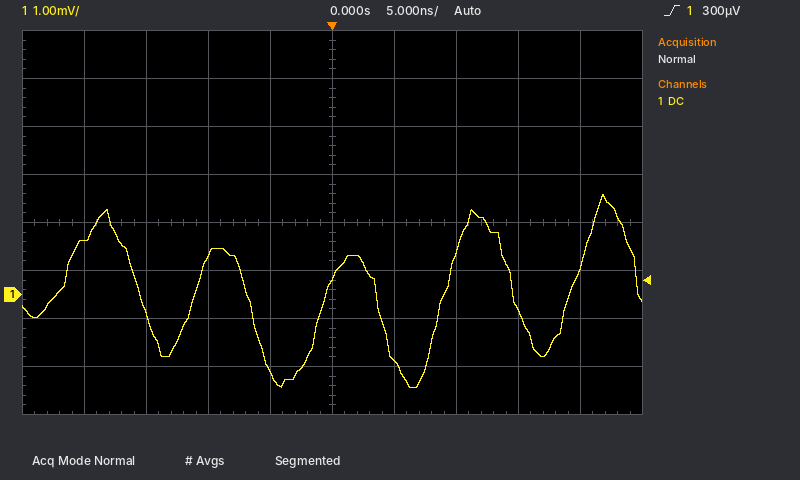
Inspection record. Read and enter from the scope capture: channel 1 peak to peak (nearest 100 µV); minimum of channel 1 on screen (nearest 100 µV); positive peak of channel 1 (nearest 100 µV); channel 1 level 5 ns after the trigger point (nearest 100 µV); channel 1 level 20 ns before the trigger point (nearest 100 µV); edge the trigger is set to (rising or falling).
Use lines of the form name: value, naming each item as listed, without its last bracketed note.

channel 1 peak to peak: 4.0 mV
minimum of channel 1 on screen: -1.9 mV
positive peak of channel 1: 2.1 mV
channel 1 level 5 ns after the trigger point: -1.4 mV
channel 1 level 20 ns before the trigger point: 1.1 mV
edge the trigger is set to: rising
